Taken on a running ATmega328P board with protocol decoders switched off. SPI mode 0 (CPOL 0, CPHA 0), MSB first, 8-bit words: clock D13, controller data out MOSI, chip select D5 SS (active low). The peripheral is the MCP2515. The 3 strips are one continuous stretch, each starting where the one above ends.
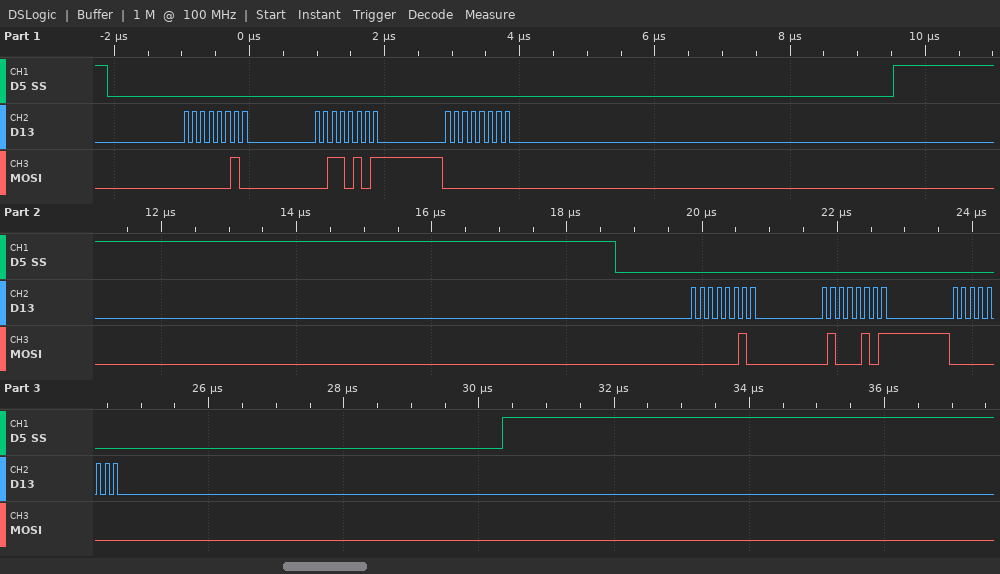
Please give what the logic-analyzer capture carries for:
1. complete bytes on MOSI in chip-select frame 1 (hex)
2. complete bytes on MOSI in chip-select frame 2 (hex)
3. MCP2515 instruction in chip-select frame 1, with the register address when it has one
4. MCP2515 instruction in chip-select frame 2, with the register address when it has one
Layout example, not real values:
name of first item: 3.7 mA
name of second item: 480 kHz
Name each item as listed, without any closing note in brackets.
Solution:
complete bytes on MOSI in chip-select frame 1: 02 35 00
complete bytes on MOSI in chip-select frame 2: 02 45 00
MCP2515 instruction in chip-select frame 1, with the register address when it has one: WRITE 0x35
MCP2515 instruction in chip-select frame 2, with the register address when it has one: WRITE 0x45
